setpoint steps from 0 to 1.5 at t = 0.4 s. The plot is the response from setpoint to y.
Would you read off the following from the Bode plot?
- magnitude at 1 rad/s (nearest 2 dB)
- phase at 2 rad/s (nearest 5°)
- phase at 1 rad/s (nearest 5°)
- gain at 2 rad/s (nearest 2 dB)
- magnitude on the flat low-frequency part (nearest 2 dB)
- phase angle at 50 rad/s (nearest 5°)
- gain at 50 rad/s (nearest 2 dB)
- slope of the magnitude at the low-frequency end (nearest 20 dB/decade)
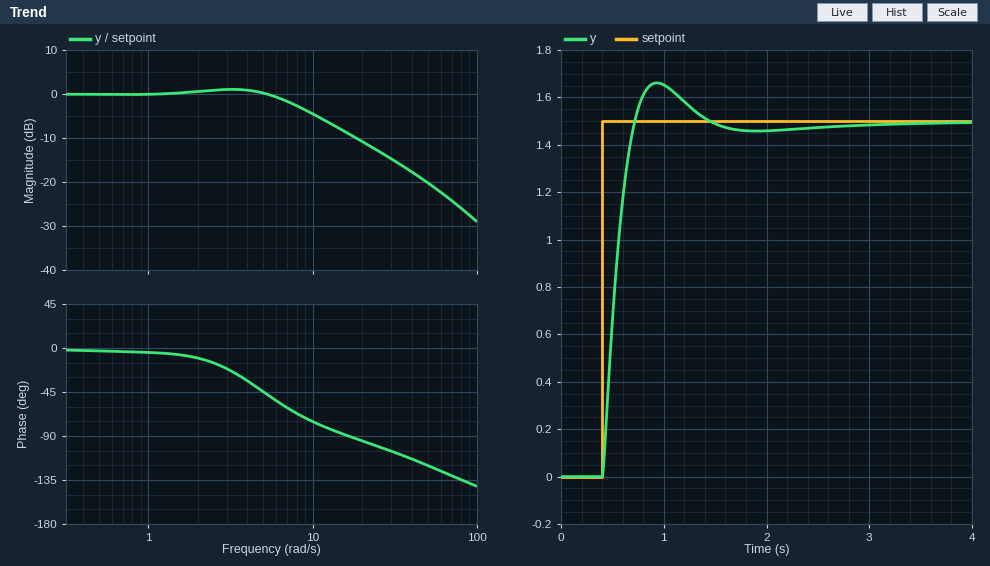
0 dB
-10°
-5°
0 dB
0 dB
-120°
-20 dB
0 dB/decade
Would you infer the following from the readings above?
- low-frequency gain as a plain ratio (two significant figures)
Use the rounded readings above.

1.0
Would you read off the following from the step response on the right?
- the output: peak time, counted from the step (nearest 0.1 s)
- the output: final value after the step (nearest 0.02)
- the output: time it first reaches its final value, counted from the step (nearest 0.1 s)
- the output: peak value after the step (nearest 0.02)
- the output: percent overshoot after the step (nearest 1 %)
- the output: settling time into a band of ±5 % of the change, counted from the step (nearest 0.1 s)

0.5 s
1.50
0.3 s
1.66
11 %
0.8 s
